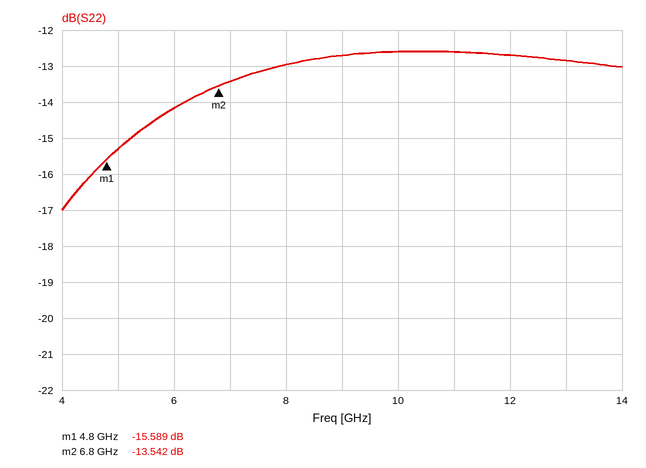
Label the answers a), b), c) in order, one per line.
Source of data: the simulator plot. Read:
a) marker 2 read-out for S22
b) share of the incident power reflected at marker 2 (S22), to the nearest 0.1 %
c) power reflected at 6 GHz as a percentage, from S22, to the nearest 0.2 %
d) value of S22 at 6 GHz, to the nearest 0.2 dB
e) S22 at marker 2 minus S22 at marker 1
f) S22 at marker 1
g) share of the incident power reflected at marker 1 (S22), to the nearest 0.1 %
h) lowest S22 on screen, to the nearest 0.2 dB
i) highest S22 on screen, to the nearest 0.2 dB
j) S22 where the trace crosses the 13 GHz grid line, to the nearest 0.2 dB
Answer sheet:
a) -13.542 dB
b) 4.4 %
c) 3.8 %
d) -14.2 dB
e) 2.047 dB
f) -15.589 dB
g) 2.8 %
h) -17.0 dB
i) -12.6 dB
j) -12.8 dB
